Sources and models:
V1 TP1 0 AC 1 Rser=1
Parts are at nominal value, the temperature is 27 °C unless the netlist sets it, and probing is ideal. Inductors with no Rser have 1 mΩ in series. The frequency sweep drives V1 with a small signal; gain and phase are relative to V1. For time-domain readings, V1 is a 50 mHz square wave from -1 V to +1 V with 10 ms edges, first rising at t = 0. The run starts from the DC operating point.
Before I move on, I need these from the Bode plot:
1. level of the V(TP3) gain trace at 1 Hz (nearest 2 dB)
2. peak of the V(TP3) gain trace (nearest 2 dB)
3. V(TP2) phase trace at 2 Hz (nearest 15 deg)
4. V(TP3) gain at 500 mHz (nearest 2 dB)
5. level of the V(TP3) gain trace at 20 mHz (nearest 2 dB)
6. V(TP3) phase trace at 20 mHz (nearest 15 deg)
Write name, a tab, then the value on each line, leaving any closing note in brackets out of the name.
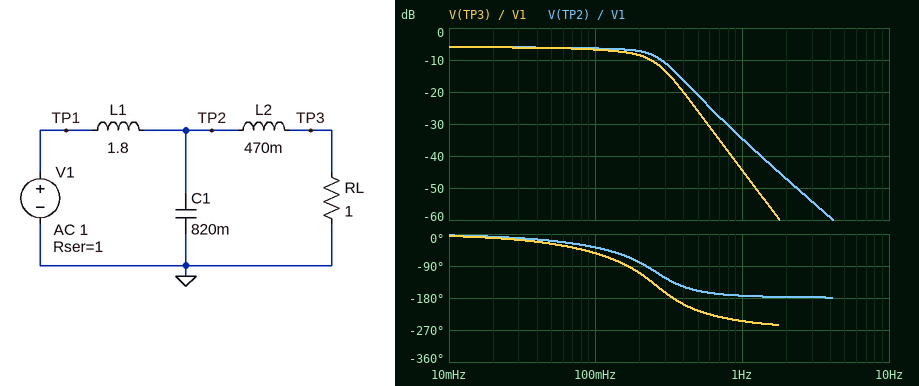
level of the V(TP3) gain trace at 1 Hz	-44 dB
peak of the V(TP3) gain trace	-6 dB
V(TP2) phase trace at 2 Hz	-180 deg
V(TP3) gain at 500 mHz	-26 dB
level of the V(TP3) gain trace at 20 mHz	-6 dB
V(TP3) phase trace at 20 mHz	-15 deg
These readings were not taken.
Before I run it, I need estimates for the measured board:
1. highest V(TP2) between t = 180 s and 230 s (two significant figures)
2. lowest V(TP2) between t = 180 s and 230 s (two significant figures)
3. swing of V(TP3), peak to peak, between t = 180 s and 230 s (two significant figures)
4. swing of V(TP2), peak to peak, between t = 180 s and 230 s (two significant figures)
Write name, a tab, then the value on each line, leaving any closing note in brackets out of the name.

highest V(TP2) between t = 180 s and 230 s	540 mV
lowest V(TP2) between t = 180 s and 230 s	-540 mV
swing of V(TP3), peak to peak, between t = 180 s and 230 s	1.0 V
swing of V(TP2), peak to peak, between t = 180 s and 230 s	1.1 V
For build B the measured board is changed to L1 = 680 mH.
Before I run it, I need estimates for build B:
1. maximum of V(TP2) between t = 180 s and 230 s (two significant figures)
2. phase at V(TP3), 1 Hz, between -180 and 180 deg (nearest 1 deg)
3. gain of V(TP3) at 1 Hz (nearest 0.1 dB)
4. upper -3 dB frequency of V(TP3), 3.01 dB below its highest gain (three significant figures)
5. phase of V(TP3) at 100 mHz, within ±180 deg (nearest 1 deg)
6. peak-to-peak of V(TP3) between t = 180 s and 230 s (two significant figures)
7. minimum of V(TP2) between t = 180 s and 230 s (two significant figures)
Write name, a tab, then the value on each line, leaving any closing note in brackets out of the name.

maximum of V(TP2) between t = 180 s and 230 s	680 mV
phase at V(TP3), 1 Hz, between -180 and 180 deg	124 deg
gain of V(TP3) at 1 Hz	-36.0 dB
upper -3 dB frequency of V(TP3), 3.01 dB below its highest gain	339 mHz
phase of V(TP3) at 100 mHz, within ±180 deg	-36 deg
peak-to-peak of V(TP3) between t = 180 s and 230 s	1.2 V
minimum of V(TP2) between t = 180 s and 230 s	-680 mV
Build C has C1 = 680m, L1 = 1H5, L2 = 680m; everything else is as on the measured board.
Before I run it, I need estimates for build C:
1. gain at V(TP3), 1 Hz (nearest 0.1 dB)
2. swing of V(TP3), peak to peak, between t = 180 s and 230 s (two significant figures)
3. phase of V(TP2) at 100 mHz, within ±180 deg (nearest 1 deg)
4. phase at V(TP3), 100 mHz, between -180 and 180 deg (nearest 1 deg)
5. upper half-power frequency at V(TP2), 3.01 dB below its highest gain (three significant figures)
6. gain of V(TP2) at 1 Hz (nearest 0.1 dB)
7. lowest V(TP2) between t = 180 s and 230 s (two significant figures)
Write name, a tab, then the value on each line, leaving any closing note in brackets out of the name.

gain at V(TP3), 1 Hz	-44.3 dB
swing of V(TP3), peak to peak, between t = 180 s and 230 s	1.1 V
phase of V(TP2) at 100 mHz, within ±180 deg	-26 deg
phase at V(TP3), 100 mHz, between -180 and 180 deg	-49 deg
upper half-power frequency at V(TP2), 3.01 dB below its highest gain	319 mHz
gain of V(TP2) at 1 Hz	-31.5 dB
lowest V(TP2) between t = 180 s and 230 s	-670 mV
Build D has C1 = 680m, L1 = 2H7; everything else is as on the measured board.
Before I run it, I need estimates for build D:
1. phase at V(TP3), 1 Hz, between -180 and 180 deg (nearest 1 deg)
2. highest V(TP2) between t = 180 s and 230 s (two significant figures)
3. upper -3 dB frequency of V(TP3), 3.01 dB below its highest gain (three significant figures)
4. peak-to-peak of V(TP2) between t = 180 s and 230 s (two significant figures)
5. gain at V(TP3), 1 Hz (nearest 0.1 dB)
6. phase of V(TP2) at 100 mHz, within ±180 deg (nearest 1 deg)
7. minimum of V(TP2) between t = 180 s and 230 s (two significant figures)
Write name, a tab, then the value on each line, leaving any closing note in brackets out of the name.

phase at V(TP3), 1 Hz, between -180 and 180 deg	114 deg
highest V(TP2) between t = 180 s and 230 s	500 mV
upper -3 dB frequency of V(TP3), 3.01 dB below its highest gain	141 mHz
peak-to-peak of V(TP2) between t = 180 s and 230 s	1.0 V
gain at V(TP3), 1 Hz	-46.3 dB
phase of V(TP2) at 100 mHz, within ±180 deg	-46 deg
minimum of V(TP2) between t = 180 s and 230 s	-500 mV
